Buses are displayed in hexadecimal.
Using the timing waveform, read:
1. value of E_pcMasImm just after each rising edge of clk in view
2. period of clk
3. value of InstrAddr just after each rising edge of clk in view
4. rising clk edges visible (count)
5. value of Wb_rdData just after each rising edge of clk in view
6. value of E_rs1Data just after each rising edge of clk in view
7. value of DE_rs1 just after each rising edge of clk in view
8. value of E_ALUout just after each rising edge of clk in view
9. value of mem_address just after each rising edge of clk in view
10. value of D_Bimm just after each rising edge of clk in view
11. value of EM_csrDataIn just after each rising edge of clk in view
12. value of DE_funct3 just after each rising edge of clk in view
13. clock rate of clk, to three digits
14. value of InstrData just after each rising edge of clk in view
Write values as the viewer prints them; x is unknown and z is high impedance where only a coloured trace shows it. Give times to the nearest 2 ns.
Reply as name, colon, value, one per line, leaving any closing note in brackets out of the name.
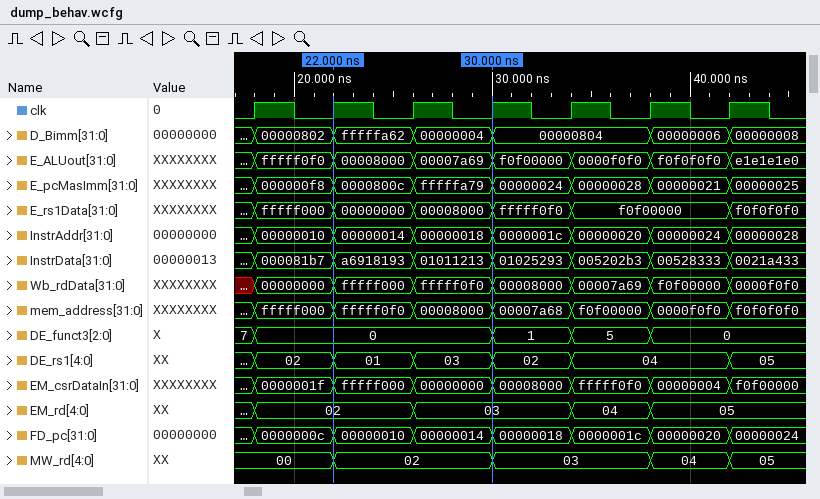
value of E_pcMasImm just after each rising edge of clk in view: 000000f8, 0000800c, fffffa79, 00000024, 00000028, 00000021, 00000025
period of clk: 4 ns
value of InstrAddr just after each rising edge of clk in view: 00000010, 00000014, 00000018, 0000001c, 00000020, 00000024, 00000028
rising clk edges visible: 7
value of Wb_rdData just after each rising edge of clk in view: 00000000, fffff000, fffff0f0, 00008000, 00007a69, f0f00000, 0000f0f0
value of E_rs1Data just after each rising edge of clk in view: fffff000, 00000000, 00008000, fffff0f0, f0f00000, f0f00000, f0f0f0f0
value of DE_rs1 just after each rising edge of clk in view: 02, 01, 03, 02, 04, 04, 05
value of E_ALUout just after each rising edge of clk in view: fffff0f0, 00008000, 00007a69, f0f00000, 0000f0f0, f0f0f0f0, e1e1e1e0
value of mem_address just after each rising edge of clk in view: fffff000, fffff0f0, 00008000, 00007a68, f0f00000, 0000f0f0, f0f0f0f0
value of D_Bimm just after each rising edge of clk in view: 00000802, fffffa62, 00000004, 00000804, 00000804, 00000006, 00000008
value of EM_csrDataIn just after each rising edge of clk in view: 0000001f, fffff000, 00000000, 00008000, fffff0f0, 00000004, f0f00000
value of DE_funct3 just after each rising edge of clk in view: 0, 0, 0, 1, 5, 0, 0
clock rate of clk, to three digits: 250 MHz
value of InstrData just after each rising edge of clk in view: 000081b7, a6918193, 01011213, 01025293, 005202b3, 00528333, 0021a433
